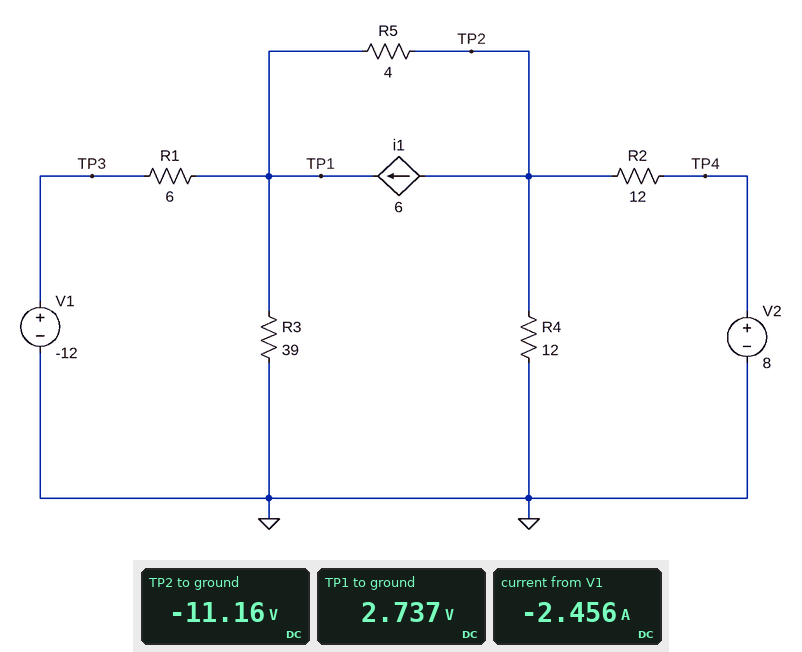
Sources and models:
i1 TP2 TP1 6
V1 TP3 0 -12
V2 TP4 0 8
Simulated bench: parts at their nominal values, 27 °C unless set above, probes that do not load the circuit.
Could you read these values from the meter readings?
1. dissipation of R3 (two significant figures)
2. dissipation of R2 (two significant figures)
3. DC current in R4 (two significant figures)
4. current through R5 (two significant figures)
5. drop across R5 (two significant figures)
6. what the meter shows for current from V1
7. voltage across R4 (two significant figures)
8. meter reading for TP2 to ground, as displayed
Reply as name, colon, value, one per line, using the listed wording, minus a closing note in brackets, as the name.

dissipation of R3: 190 mW
dissipation of R2: 31 W
DC current in R4: 930 mA
current through R5: 3.5 A
drop across R5: 14 V
what the meter shows for current from V1: -2.456 A
voltage across R4: 11 V
meter reading for TP2 to ground, as displayed: -11.16 V
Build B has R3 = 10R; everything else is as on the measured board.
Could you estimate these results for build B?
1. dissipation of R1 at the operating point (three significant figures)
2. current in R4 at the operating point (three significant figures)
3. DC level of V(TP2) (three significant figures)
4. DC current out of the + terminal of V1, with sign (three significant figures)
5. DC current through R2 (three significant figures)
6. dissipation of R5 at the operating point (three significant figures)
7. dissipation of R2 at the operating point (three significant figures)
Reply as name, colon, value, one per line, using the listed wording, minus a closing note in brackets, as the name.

dissipation of R1 at the operating point: 33.5 W
current in R4 at the operating point: 958 mA
DC level of V(TP2): -11.5 V
DC current out of the + terminal of V1, with sign: -2.36 A
DC current through R2: 1.62 A
dissipation of R5 at the operating point: 46.7 W
dissipation of R2 at the operating point: 31.7 W
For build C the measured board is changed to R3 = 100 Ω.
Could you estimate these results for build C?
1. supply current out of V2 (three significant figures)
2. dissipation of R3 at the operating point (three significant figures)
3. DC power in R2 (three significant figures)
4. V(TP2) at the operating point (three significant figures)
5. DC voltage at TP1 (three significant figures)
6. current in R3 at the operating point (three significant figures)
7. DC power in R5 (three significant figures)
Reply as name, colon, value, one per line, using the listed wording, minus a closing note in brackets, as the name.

supply current out of V2: 1.59 A
dissipation of R3 at the operating point: 83.6 mW
DC power in R2: 30.3 W
V(TP2) at the operating point: -11.1 V
DC voltage at TP1: 2.89 V
current in R3 at the operating point: 28.9 mA
DC power in R5: 48.7 W
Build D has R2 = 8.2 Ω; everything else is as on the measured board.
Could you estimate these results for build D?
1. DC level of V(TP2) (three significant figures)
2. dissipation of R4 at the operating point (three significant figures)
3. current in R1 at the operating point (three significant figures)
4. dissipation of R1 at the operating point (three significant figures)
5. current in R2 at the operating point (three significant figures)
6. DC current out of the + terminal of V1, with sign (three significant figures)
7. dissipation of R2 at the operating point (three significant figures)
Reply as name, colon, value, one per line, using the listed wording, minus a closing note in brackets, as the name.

DC level of V(TP2): -8.80 V
dissipation of R4 at the operating point: 6.46 W
current in R1 at the operating point: 2.68 A
dissipation of R1 at the operating point: 43.0 W
current in R2 at the operating point: 2.05 A
DC current out of the + terminal of V1, with sign: -2.68 A
dissipation of R2 at the operating point: 34.4 W
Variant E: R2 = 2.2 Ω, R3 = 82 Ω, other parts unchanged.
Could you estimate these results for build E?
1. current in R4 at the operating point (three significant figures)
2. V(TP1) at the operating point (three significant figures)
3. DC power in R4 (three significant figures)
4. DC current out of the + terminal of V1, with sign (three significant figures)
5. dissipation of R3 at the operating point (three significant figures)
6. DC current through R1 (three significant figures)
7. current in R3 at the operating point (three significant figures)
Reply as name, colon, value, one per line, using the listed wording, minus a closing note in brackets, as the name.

current in R4 at the operating point: 4.14 mA
V(TP1) at the operating point: 9.30 V
DC power in R4: 205 µW
DC current out of the + terminal of V1, with sign: -3.55 A
dissipation of R3 at the operating point: 1.05 W
DC current through R1: 3.55 A
current in R3 at the operating point: 113 mA
